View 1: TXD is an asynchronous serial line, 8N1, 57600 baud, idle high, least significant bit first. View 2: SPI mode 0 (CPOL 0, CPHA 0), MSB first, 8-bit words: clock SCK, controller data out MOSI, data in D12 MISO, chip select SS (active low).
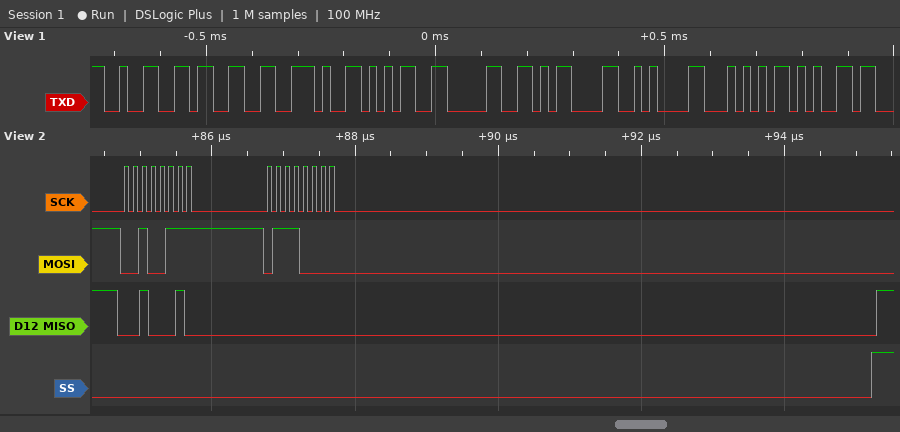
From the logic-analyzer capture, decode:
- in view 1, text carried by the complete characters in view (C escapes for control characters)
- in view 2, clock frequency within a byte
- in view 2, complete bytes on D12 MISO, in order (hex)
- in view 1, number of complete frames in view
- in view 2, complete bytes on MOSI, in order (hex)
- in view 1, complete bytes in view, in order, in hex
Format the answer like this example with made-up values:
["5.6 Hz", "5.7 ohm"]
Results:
["\"23.50\\r\\nTe\"", "8 MHz", "0x22 0x00", "9", "0x27 0x70", "32 33 2E 35 30 0D 0A 54 65"]
